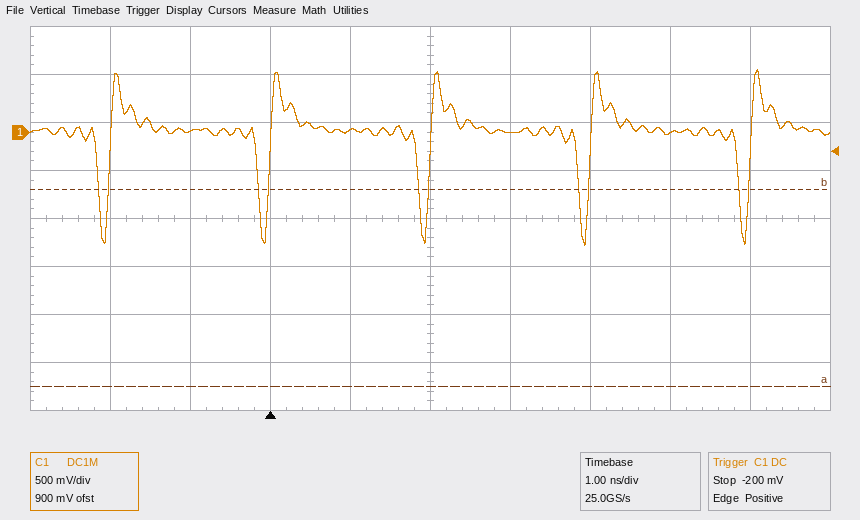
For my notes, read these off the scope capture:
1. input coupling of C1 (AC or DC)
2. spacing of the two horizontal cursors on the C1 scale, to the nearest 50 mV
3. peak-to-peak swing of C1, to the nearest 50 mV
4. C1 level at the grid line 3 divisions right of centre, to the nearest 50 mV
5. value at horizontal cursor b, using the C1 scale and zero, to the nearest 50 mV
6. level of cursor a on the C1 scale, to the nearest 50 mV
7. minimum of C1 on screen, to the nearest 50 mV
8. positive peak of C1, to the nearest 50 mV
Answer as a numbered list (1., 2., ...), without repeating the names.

1. DC
2. 2.05 V
3. 1.85 V
4. 0 mV
5. -600 mV
6. -2.65 V
7. -1.20 V
8. 650 mV
